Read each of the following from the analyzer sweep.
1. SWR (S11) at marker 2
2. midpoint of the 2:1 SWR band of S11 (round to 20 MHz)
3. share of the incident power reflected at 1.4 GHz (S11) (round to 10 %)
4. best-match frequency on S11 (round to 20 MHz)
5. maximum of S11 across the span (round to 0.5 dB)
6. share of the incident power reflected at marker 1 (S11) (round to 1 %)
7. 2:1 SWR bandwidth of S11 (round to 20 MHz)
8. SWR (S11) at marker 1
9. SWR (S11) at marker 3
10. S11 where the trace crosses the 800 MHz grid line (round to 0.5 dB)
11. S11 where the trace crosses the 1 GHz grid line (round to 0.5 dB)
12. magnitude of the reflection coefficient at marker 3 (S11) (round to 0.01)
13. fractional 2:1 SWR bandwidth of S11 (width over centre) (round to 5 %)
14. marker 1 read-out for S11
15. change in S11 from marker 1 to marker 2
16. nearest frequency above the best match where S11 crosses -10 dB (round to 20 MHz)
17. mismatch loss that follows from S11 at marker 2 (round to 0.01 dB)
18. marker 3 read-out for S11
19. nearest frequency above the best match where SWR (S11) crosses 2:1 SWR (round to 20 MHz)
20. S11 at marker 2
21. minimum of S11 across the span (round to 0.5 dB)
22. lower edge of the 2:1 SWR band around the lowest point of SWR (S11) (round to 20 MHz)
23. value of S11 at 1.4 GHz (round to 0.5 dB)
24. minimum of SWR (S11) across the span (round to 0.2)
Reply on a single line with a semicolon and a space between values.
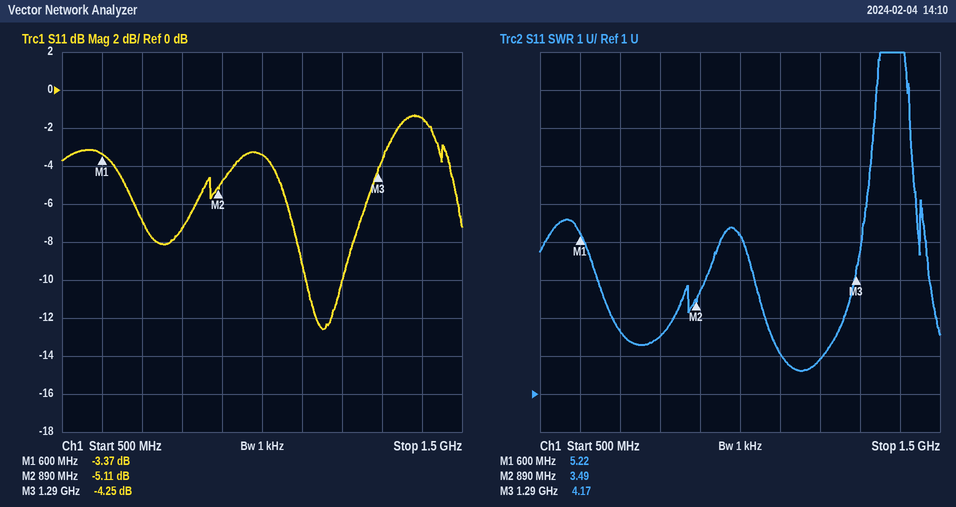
3.49; 1.16 GHz; 70 %; 1.16 GHz; -1.5 dB; 46 %; 100 MHz; 5.22; 4.17; -7.5 dB; -3.5 dB; 0.61; 10 %; -3.37 dB; -1.74 dB; 1.20 GHz; 1.60 dB; -4.25 dB; 1.20 GHz; -5.11 dB; -12.5 dB; 1.10 GHz; -1.5 dB; 1.6
